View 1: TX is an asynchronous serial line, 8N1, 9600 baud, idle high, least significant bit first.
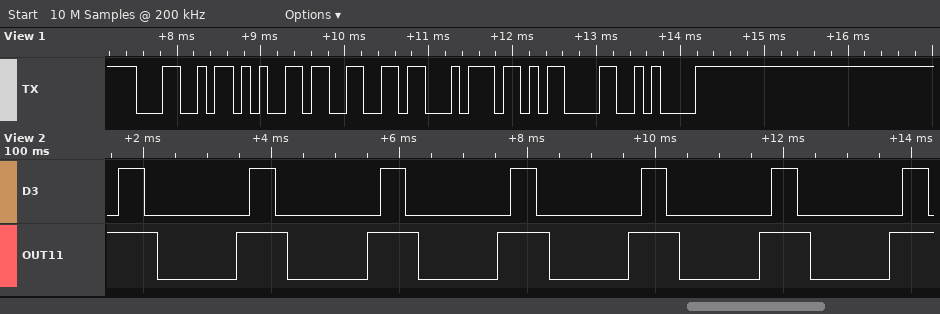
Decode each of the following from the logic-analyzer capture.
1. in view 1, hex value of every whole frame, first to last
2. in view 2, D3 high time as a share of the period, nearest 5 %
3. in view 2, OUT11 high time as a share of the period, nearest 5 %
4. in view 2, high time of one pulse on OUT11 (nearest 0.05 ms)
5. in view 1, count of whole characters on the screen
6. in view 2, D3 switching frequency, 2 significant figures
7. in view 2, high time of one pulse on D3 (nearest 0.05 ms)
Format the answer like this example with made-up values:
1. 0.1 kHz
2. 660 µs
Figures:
1. 0x4C 0x65 0x66 0x74 0x0D 0x0A
2. 20 %
3. 40 %
4. 0.80 ms
5. 6
6. 490 Hz
7. 0.40 ms
